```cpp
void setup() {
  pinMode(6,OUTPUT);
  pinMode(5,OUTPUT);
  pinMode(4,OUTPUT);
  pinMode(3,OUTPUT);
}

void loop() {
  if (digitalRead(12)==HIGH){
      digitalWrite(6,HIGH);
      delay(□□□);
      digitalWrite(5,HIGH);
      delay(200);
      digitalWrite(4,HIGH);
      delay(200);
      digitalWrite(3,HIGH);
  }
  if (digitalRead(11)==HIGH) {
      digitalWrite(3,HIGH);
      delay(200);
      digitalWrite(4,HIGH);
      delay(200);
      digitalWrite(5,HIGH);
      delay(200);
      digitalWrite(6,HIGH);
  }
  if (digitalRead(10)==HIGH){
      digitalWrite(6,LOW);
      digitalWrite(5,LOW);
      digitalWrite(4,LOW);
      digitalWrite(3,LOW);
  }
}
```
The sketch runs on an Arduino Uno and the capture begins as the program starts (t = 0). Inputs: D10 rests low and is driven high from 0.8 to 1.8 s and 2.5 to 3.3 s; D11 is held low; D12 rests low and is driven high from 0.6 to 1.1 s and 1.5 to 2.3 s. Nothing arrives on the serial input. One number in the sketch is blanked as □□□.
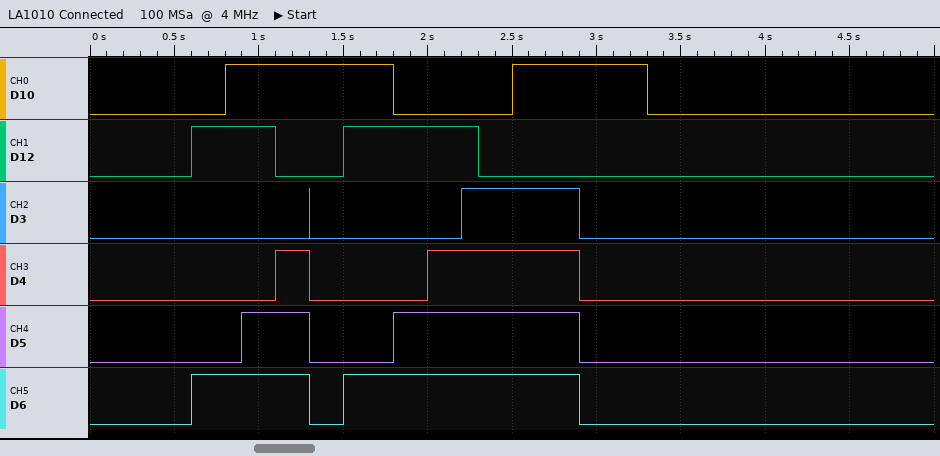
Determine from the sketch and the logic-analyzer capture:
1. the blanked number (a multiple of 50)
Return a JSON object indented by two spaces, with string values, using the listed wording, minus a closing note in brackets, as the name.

{
  "the blanked number": "300"
}
